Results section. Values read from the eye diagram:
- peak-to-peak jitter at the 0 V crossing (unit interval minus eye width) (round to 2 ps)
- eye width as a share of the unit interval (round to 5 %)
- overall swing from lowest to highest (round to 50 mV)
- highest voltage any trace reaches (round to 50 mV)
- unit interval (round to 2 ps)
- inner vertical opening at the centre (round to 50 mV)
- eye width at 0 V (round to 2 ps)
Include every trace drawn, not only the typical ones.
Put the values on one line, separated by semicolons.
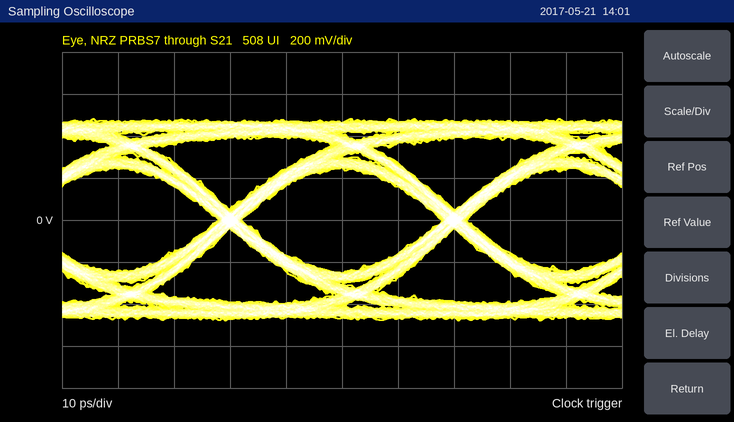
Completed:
4 ps; 90 %; 950 mV; 500 mV; 40 ps; 500 mV; 36 ps
